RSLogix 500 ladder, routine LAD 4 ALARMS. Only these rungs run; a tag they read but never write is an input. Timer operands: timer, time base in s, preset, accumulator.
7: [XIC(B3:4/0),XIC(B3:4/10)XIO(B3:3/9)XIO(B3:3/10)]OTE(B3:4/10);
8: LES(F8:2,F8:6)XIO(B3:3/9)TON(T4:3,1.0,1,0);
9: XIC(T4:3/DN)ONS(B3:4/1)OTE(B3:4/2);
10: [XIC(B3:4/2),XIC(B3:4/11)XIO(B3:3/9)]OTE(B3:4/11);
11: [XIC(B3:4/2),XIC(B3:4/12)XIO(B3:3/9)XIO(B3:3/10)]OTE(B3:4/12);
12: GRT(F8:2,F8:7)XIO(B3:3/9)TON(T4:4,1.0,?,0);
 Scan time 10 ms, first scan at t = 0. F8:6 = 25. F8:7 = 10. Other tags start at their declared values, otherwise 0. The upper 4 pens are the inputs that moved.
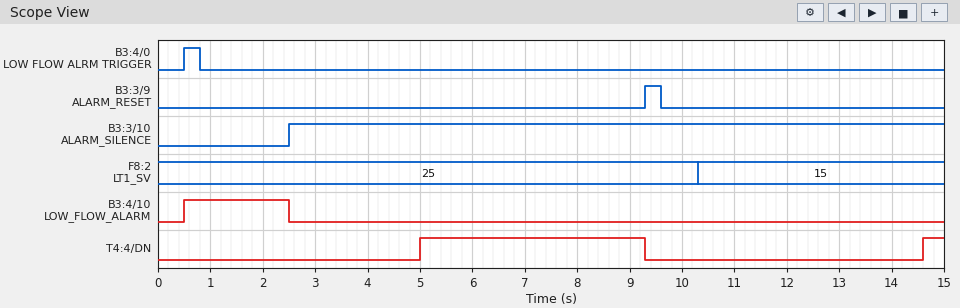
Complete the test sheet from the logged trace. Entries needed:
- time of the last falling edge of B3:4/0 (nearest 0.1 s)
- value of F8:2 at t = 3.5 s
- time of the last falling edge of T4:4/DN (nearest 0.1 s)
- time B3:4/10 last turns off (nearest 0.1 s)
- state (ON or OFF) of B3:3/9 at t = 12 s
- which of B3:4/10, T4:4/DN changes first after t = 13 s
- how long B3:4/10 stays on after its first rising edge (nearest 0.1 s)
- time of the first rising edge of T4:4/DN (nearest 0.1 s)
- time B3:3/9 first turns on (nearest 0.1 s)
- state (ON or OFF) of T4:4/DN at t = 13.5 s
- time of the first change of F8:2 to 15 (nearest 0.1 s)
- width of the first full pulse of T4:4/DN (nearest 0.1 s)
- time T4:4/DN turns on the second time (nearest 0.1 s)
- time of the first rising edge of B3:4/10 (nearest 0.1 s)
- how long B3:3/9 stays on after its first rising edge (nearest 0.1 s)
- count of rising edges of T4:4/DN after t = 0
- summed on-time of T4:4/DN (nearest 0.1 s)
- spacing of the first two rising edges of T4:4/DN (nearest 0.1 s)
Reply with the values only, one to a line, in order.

0.8 s
25
9.3 s
2.5 s
OFF
T4:4/DN
2.0 s
5.0 s
9.3 s
OFF
10.3 s
4.3 s
14.6 s
0.5 s
0.3 s
2
4.7 s
9.6 s
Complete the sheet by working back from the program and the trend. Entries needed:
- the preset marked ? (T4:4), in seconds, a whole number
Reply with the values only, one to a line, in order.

5 s
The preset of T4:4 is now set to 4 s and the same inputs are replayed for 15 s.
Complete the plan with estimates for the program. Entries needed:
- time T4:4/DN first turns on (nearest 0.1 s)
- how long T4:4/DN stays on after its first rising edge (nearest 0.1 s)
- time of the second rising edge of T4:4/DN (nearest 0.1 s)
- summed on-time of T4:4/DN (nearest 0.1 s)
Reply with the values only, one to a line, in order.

4.0 s
5.3 s
13.6 s
6.7 s
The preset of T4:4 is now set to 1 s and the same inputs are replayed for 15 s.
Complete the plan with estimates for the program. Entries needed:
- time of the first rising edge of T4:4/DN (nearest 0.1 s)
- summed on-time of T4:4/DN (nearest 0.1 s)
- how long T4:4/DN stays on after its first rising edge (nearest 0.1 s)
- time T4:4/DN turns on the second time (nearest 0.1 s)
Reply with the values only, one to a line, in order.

1.0 s
12.7 s
8.3 s
10.6 s
